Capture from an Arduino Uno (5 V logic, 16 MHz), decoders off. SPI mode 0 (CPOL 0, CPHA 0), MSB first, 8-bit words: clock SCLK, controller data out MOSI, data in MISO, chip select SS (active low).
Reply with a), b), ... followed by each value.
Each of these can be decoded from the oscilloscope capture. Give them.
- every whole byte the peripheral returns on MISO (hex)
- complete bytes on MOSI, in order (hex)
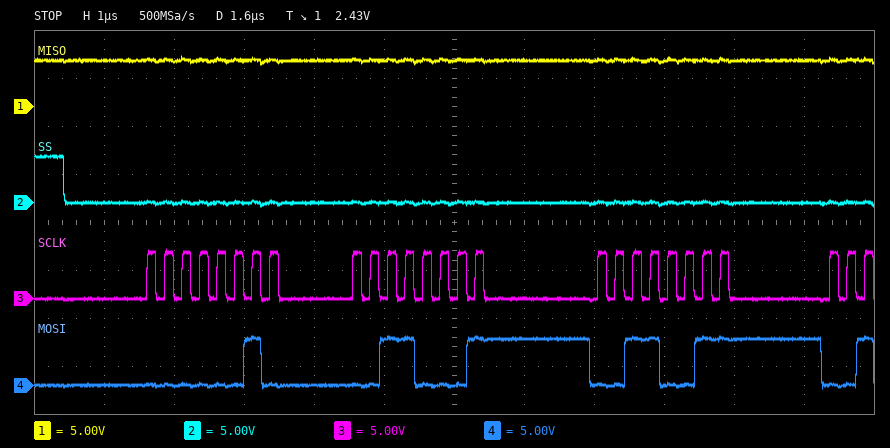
a) FF FF FF
b) 02 31 33
